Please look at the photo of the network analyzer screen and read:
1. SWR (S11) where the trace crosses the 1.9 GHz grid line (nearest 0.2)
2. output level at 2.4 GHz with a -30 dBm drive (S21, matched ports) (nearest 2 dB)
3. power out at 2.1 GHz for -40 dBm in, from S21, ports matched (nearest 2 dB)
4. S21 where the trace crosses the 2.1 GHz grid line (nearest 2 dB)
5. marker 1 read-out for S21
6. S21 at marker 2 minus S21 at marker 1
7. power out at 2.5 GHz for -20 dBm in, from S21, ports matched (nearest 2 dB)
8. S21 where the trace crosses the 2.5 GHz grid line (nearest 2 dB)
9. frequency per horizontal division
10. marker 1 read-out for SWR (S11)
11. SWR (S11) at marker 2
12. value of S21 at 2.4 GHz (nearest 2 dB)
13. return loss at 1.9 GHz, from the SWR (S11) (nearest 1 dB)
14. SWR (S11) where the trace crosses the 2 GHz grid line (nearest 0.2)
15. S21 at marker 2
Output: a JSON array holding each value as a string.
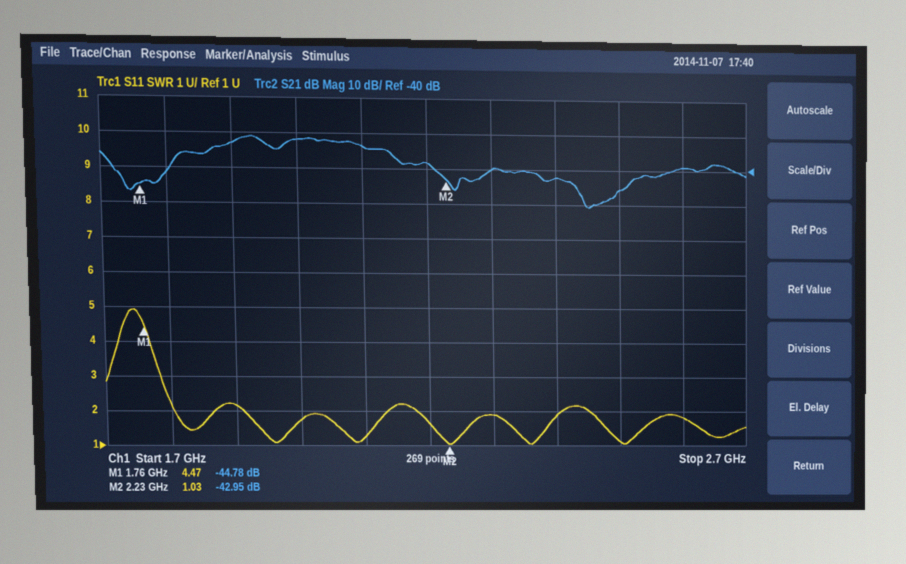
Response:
["2.2", "-72 dBm", "-74 dBm", "-34 dB", "-44.78 dB", "1.83 dB", "-66 dBm", "-46 dB", "100 MHz", "4.47", "1.03", "-42 dB", "9 dB", "1.8", "-42.95 dB"]
